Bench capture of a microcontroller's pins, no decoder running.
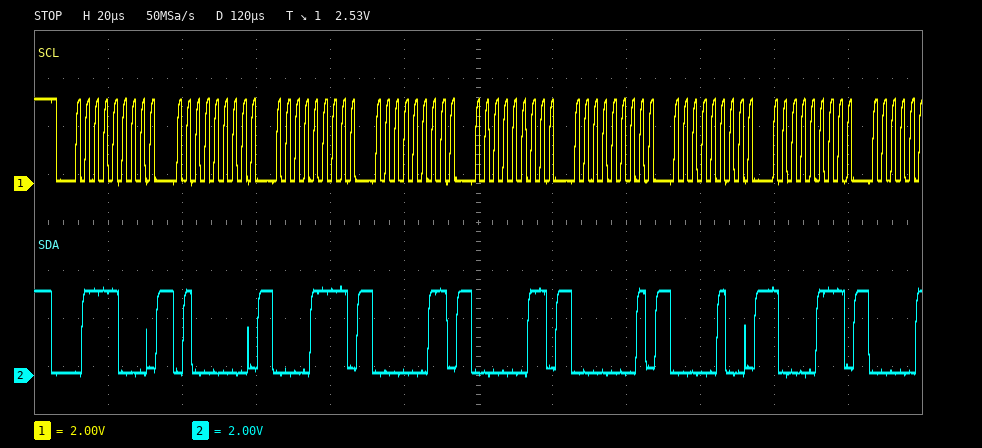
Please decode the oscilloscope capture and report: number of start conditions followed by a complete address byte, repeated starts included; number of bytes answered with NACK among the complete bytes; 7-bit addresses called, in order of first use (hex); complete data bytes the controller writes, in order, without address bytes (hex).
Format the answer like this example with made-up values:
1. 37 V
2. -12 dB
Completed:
1. 1
2. 0
3. 0x3C
4. 40 0F 03 03 01 04 87
